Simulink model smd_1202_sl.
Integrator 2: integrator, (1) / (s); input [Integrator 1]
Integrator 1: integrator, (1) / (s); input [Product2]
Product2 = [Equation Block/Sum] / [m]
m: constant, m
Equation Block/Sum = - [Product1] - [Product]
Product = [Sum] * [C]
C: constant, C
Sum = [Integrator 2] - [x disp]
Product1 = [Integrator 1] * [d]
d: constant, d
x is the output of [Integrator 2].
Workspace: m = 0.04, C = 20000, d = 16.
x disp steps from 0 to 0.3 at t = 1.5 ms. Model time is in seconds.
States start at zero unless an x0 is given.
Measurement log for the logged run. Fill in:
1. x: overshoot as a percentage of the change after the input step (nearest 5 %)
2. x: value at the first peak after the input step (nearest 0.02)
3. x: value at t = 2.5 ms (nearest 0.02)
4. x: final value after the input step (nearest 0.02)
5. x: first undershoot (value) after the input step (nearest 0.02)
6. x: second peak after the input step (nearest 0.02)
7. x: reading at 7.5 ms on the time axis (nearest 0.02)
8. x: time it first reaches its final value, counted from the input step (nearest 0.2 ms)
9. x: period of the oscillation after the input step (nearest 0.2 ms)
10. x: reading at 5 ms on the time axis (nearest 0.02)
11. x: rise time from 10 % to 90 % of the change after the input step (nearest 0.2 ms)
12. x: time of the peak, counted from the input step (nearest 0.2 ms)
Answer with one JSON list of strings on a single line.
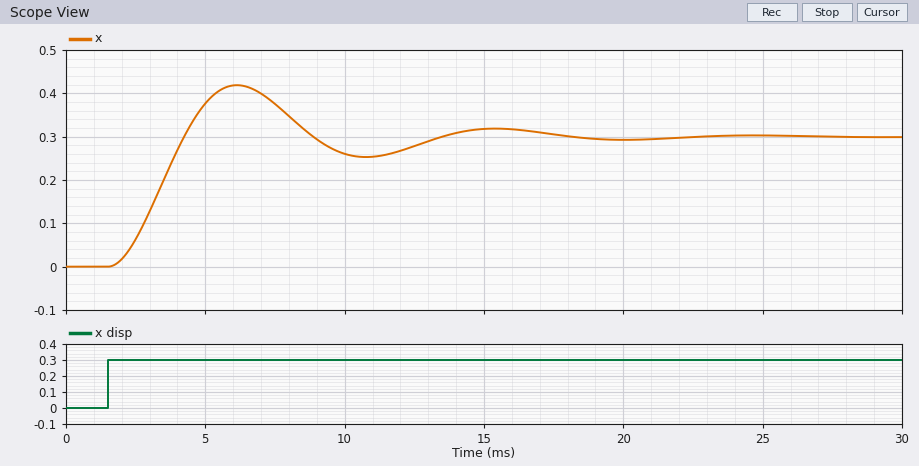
["40 %", "0.42", "0.06", "0.30", "0.26", "0.32", "0.38", "2.8 ms", "9.2 ms", "0.38", "1.8 ms", "4.6 ms"]
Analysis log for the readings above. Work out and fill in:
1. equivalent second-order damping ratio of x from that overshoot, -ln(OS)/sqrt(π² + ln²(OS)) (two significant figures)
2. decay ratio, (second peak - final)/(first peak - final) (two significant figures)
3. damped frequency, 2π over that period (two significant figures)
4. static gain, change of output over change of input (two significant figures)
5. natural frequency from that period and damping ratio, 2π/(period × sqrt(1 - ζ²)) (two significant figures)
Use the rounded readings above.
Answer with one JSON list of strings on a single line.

["0.28", "0.17", "0.68 rad/ms", "1.0", "0.71 rad/ms"]
